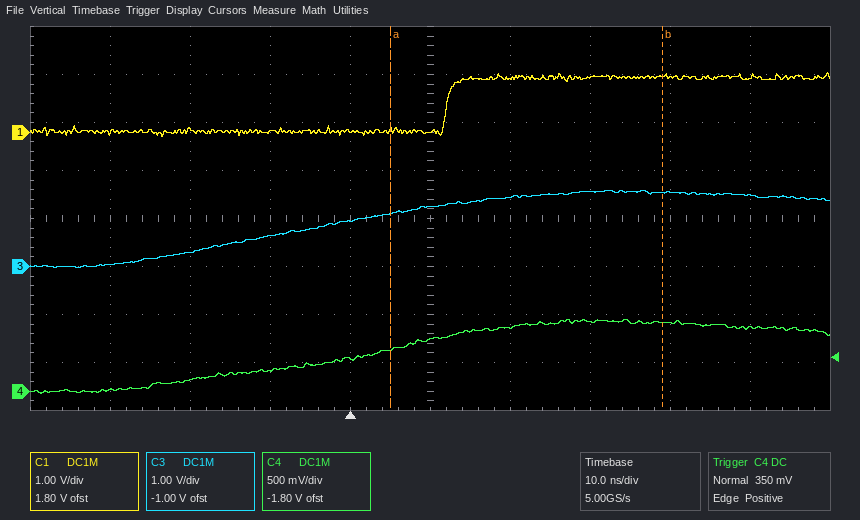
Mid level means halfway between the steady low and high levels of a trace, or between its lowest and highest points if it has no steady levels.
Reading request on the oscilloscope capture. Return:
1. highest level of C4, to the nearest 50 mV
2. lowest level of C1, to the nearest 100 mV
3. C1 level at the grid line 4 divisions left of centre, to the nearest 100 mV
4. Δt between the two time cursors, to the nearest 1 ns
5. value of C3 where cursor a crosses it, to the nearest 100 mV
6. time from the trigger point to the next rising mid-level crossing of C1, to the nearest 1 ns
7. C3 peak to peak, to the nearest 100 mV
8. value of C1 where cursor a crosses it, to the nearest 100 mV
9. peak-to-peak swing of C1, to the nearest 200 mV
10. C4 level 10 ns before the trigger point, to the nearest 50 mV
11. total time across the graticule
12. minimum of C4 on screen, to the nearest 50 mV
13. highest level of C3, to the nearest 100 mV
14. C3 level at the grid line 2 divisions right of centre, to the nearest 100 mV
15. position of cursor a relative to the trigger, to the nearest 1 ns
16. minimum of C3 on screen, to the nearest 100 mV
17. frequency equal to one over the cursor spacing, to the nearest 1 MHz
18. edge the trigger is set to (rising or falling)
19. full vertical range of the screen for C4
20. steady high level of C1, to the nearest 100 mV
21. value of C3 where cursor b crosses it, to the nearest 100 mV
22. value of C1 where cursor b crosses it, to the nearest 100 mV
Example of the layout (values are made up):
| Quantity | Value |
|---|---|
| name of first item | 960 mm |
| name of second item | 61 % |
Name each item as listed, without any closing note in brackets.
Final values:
| Quantity | Value |
|---|---|
| highest level of C4, to the nearest 50 mV | 750 mV |
| lowest level of C1, to the nearest 100 mV | -100 mV |
| C1 level at the grid line 4 divisions left of centre, to the nearest 100 mV | 0.0 V |
| Δt between the two time cursors, to the nearest 1 ns | 34 ns |
| value of C3 where cursor a crosses it, to the nearest 100 mV | 1.1 V |
| time from the trigger point to the next rising mid-level crossing of C1, to the nearest 1 ns | 12 ns |
| C3 peak to peak, to the nearest 100 mV | 1.6 V |
| value of C1 where cursor a crosses it, to the nearest 100 mV | 0.0 V |
| peak-to-peak swing of C1, to the nearest 200 mV | 1.4 V |
| C4 level 10 ns before the trigger point, to the nearest 50 mV | 200 mV |
| total time across the graticule | 100 ns |
| minimum of C4 on screen, to the nearest 50 mV | 0 mV |
| highest level of C3, to the nearest 100 mV | 1.6 V |
| C3 level at the grid line 2 divisions right of centre, to the nearest 100 mV | 1.6 V |
| position of cursor a relative to the trigger, to the nearest 1 ns | +5 ns |
| minimum of C3 on screen, to the nearest 100 mV | 0.0 V |
| frequency equal to one over the cursor spacing, to the nearest 1 MHz | 29 MHz |
| edge the trigger is set to | rising |
| full vertical range of the screen for C4 | 4 V |
| steady high level of C1, to the nearest 100 mV | 1.1 V |
| value of C3 where cursor b crosses it, to the nearest 100 mV | 1.5 V |
| value of C1 where cursor b crosses it, to the nearest 100 mV | 1.2 V |
